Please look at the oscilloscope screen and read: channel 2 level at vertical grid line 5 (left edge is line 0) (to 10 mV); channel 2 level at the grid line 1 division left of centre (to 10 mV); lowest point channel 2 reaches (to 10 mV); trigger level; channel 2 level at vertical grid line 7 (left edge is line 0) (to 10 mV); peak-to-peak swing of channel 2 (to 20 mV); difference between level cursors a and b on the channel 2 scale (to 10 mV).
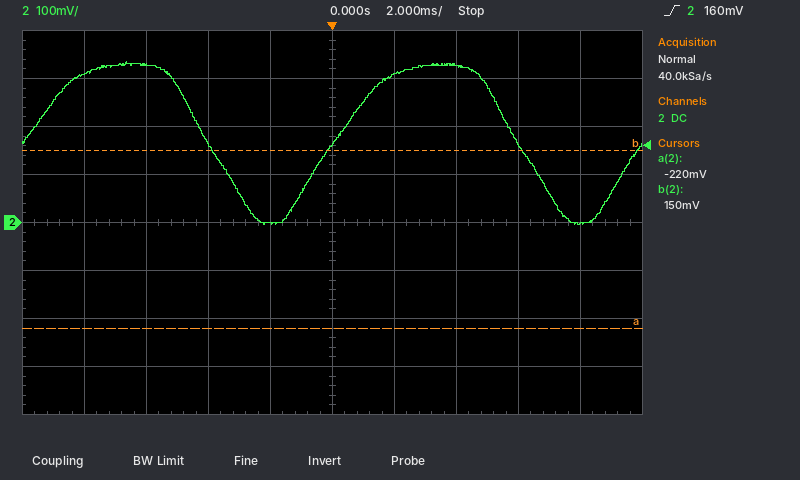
160 mV
0 mV
0 mV
160 mV
330 mV
340 mV
370 mV
